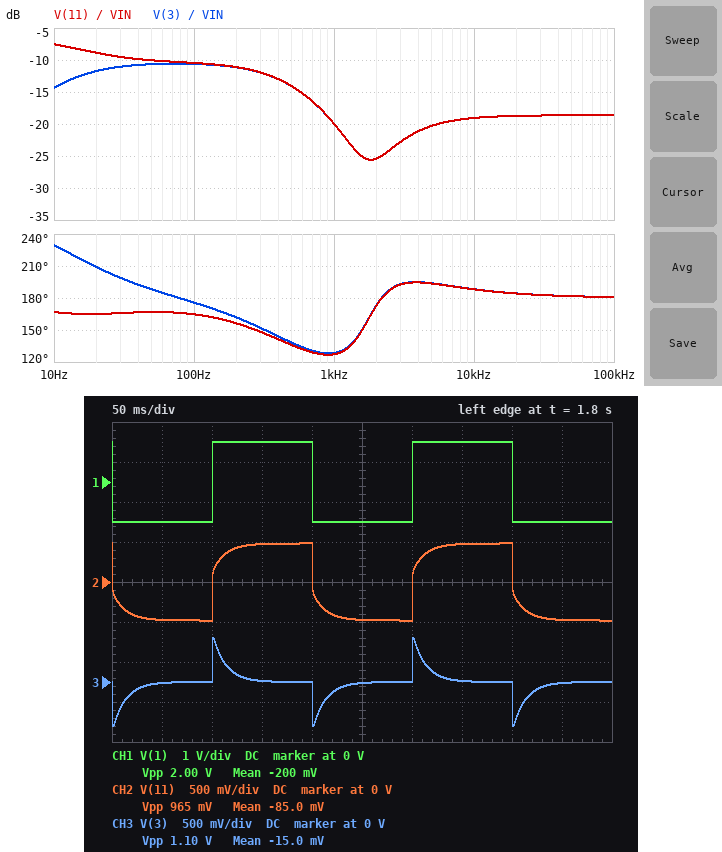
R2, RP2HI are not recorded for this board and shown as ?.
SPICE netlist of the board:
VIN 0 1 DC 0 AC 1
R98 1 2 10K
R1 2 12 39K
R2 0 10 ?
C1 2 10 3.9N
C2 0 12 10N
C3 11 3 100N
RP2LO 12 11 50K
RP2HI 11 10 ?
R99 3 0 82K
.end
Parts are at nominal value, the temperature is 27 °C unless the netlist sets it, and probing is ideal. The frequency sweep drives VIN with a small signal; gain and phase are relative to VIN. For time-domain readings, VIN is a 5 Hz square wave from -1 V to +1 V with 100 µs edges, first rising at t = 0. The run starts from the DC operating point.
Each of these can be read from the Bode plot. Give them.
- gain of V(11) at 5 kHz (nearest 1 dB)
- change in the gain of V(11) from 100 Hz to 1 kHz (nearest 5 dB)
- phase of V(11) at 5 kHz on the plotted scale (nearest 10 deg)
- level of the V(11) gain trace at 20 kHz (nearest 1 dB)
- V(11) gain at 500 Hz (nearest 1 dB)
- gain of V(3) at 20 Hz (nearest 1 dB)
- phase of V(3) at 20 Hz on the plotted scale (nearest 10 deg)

-20 dB
-10 dB
190 deg
-19 dB
-14 dB
-12 dB
210 deg
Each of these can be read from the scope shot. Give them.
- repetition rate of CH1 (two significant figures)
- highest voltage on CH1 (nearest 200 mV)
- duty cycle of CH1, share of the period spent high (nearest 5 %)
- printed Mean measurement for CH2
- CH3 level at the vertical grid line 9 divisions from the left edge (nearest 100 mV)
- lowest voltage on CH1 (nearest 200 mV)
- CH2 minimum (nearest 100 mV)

5.0 Hz
1.0 V
50 %
-85.0 mV
0 V
-1.0 V
-500 mV
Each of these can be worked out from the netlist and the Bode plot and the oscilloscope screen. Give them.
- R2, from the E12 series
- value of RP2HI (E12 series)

10 kΩ
82 kΩ
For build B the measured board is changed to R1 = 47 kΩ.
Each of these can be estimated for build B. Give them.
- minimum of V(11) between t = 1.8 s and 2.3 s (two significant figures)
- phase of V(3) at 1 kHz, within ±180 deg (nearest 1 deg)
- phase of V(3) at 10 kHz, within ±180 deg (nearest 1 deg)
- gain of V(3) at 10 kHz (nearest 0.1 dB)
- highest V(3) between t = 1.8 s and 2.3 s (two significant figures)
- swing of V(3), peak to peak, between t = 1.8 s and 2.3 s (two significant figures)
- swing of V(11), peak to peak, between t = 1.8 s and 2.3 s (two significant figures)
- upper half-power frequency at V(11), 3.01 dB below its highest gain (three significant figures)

-460 mV
130 deg
-171 deg
-18.9 dB
520 mV
1.0 V
920 mV
25.0 Hz
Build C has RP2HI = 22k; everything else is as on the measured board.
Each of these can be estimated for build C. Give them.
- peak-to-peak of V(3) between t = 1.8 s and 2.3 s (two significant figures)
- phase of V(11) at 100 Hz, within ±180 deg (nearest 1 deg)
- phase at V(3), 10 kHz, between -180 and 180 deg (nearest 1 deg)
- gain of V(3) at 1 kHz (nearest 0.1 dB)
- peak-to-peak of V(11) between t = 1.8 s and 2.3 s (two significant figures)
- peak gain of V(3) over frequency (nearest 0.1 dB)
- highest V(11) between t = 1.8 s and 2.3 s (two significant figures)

680 mV
170 deg
-168 deg
-23.0 dB
490 mV
-12.4 dB
240 mV
